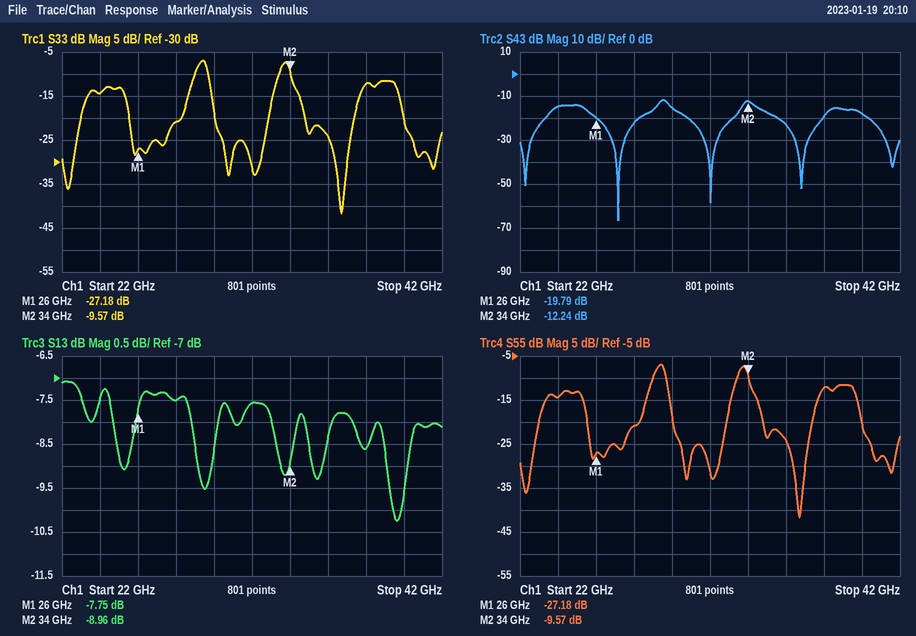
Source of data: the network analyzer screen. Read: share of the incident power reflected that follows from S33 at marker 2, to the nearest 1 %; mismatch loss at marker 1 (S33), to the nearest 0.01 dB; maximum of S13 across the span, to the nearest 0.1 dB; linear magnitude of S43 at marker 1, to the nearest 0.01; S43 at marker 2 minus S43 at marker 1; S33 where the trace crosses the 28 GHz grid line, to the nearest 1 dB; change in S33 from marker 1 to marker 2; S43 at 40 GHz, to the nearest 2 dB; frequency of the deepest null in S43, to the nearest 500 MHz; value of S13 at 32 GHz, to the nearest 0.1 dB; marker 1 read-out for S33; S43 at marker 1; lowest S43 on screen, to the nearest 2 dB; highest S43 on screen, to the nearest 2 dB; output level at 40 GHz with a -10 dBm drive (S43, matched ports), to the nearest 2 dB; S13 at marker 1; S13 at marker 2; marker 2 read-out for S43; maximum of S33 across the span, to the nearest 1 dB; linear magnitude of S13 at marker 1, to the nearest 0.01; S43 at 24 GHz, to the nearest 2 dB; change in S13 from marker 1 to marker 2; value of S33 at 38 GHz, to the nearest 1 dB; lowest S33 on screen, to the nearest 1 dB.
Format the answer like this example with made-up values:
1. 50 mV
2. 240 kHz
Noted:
1. 11 %
2. 0.01 dB
3. -7.1 dB
4. 0.10
5. 7.55 dB
6. -21 dB
7. 17.61 dB
8. -18 dB
9. 27.0 GHz
10. -7.6 dB
11. -27.18 dB
12. -19.79 dB
13. -66 dB
14. -12 dB
15. -28 dBm
16. -7.75 dB
17. -8.96 dB
18. -12.24 dB
19. -7 dB
20. 0.41
21. -14 dB
22. -1.21 dB
23. -12 dB
24. -42 dB
